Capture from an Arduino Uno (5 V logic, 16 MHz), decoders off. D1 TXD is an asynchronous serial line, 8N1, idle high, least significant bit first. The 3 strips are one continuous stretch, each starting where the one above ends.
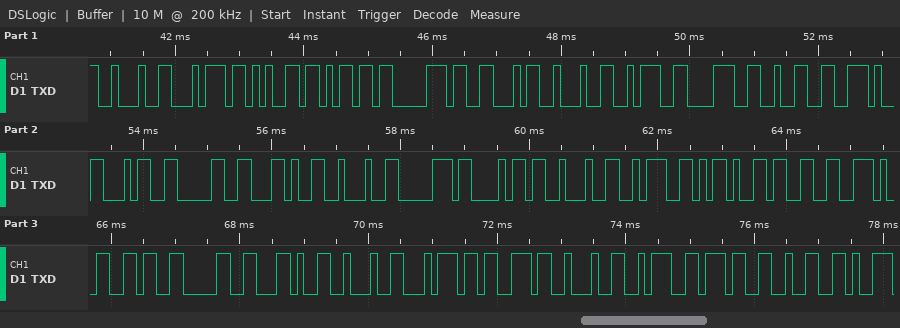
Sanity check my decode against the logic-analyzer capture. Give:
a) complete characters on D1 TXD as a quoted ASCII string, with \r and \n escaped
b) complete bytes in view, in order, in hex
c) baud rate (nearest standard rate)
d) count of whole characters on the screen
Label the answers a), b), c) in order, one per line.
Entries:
a) "\"tempF\":82.40,\"ph\":-3.60,\"ts\":72"
b) 22 74 65 6D 70 46 22 3A 38 32 2E 34 30 2C 22 70 68 22 3A 2D 33 2E 36 30 2C 22 74 73 22 3A 37 32
c) 9600 baud
d) 32
